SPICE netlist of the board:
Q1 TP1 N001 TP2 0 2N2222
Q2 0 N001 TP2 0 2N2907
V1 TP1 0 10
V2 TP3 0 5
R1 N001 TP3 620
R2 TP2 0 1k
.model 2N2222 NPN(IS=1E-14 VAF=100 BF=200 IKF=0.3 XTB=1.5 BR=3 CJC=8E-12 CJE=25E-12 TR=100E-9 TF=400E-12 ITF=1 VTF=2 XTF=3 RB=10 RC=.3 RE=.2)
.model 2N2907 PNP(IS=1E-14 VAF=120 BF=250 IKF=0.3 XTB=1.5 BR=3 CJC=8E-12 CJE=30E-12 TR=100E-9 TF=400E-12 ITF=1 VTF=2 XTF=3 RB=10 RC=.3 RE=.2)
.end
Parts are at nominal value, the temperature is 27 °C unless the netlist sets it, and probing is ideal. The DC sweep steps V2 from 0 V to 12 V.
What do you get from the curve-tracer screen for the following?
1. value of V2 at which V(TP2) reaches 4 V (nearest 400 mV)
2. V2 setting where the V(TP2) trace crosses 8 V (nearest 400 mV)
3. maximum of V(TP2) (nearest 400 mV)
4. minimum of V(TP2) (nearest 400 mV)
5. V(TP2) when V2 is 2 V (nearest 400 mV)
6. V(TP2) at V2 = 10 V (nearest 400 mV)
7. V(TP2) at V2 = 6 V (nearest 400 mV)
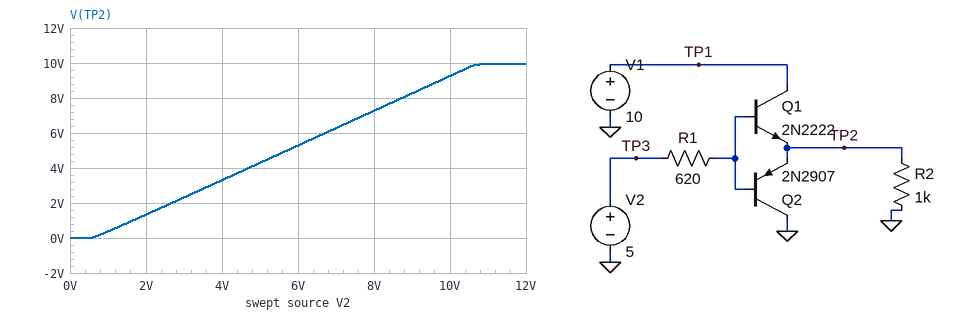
4.8 V
8.8 V
10.0 V
0 V
1.2 V
9.2 V
5.2 V
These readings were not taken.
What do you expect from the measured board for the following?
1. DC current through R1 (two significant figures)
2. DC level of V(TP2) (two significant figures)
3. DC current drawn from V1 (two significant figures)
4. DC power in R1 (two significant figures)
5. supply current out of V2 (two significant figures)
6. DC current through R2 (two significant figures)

21 µA
4.3 V
4.3 mA
260 nW
21 µA
4.3 mA
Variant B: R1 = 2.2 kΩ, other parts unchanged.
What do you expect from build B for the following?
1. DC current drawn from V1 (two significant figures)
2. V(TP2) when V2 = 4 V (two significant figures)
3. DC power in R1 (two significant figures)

4.2 mA
3.3 V
920 nW
